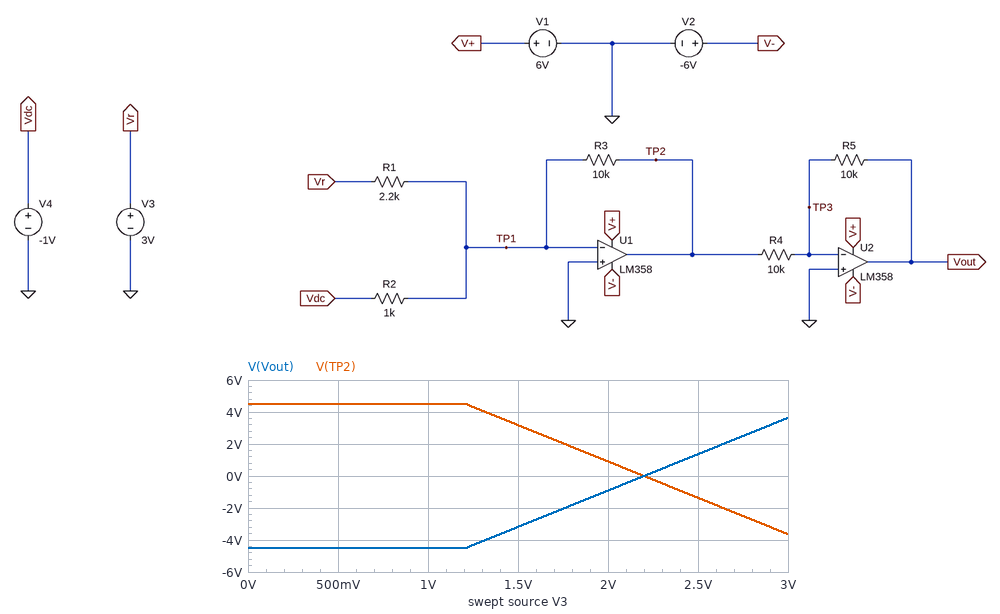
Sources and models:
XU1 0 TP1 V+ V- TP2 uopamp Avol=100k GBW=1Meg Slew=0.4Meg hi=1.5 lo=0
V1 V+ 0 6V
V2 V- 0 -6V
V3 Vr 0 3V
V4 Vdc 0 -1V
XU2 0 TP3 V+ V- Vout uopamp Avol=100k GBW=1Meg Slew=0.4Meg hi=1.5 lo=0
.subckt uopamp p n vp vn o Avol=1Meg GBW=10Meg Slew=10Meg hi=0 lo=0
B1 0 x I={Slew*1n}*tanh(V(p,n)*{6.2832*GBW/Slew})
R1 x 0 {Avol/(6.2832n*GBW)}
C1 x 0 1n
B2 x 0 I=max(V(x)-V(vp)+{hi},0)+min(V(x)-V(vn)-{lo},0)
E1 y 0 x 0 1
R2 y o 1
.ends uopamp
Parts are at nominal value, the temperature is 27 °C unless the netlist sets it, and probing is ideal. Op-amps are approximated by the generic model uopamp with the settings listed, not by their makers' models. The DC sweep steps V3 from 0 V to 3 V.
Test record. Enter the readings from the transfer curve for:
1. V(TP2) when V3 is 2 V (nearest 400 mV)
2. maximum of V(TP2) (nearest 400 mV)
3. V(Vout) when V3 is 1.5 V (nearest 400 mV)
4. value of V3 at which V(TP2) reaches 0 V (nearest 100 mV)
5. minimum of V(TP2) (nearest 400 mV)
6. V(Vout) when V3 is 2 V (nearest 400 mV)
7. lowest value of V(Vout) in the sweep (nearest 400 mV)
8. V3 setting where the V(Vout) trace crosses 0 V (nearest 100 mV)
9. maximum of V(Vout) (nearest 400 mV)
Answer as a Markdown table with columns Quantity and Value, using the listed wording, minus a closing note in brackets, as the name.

| Quantity | Value |
|---|---|
| V(TP2) when V3 is 2 V | 800 mV |
| maximum of V(TP2) | 4.4 V |
| V(Vout) when V3 is 1.5 V | -3.2 V |
| value of V3 at which V(TP2) reaches 0 V | 2.2 V |
| minimum of V(TP2) | -3.6 V |
| V(Vout) when V3 is 2 V | -800 mV |
| lowest value of V(Vout) in the sweep | -4.4 V |
| V3 setting where the V(Vout) trace crosses 0 V | 2.2 V |
| maximum of V(Vout) | 3.6 V |
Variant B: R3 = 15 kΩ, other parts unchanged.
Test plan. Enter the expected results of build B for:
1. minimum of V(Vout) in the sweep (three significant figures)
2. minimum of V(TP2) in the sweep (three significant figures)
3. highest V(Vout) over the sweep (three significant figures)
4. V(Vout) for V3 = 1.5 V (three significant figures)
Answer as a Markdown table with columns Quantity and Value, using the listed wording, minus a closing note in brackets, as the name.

| Quantity | Value |
|---|---|
| minimum of V(Vout) in the sweep | -4.50 V |
| minimum of V(TP2) in the sweep | -5.45 V |
| highest V(Vout) over the sweep | 4.50 V |
| V(Vout) for V3 = 1.5 V | -4.50 V |
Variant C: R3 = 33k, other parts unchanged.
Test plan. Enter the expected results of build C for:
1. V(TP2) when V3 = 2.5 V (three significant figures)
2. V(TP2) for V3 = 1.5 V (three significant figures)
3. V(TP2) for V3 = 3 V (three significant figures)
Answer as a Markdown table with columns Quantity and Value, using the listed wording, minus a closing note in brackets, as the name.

| Quantity | Value |
|---|---|
| V(TP2) when V3 = 2.5 V | -4.50 V |
| V(TP2) for V3 = 1.5 V | 4.50 V |
| V(TP2) for V3 = 3 V | -6.00 V |
